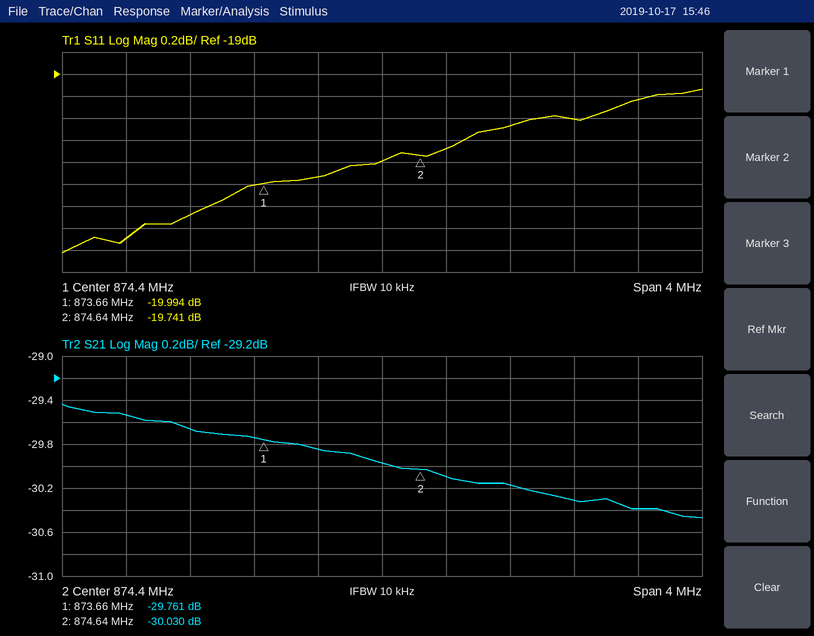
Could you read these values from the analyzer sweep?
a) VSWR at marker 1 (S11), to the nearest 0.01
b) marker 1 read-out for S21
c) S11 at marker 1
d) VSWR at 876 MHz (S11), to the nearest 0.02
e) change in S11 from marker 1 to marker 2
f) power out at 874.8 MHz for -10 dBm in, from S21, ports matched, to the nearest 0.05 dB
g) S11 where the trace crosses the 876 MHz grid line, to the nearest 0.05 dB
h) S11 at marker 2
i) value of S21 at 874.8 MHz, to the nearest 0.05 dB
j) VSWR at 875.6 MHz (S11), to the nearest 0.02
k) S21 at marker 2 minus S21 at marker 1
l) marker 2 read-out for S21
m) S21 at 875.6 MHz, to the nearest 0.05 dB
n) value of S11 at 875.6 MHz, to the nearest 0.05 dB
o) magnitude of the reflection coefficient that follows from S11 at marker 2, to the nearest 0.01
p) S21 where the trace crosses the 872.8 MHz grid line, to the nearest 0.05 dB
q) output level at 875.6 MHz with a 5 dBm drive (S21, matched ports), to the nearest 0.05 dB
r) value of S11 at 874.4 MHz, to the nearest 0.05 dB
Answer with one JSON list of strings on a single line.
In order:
["1.22", "-29.761 dB", "-19.994 dB", "1.24", "0.253 dB", "-40.10 dBm", "-19.25 dB", "-19.741 dB", "-30.10 dB", "1.24", "-0.269 dB", "-30.030 dB", "-30.30 dB", "-19.40 dB", "0.10", "-29.55 dB", "-25.30 dBm", "-19.80 dB"]
